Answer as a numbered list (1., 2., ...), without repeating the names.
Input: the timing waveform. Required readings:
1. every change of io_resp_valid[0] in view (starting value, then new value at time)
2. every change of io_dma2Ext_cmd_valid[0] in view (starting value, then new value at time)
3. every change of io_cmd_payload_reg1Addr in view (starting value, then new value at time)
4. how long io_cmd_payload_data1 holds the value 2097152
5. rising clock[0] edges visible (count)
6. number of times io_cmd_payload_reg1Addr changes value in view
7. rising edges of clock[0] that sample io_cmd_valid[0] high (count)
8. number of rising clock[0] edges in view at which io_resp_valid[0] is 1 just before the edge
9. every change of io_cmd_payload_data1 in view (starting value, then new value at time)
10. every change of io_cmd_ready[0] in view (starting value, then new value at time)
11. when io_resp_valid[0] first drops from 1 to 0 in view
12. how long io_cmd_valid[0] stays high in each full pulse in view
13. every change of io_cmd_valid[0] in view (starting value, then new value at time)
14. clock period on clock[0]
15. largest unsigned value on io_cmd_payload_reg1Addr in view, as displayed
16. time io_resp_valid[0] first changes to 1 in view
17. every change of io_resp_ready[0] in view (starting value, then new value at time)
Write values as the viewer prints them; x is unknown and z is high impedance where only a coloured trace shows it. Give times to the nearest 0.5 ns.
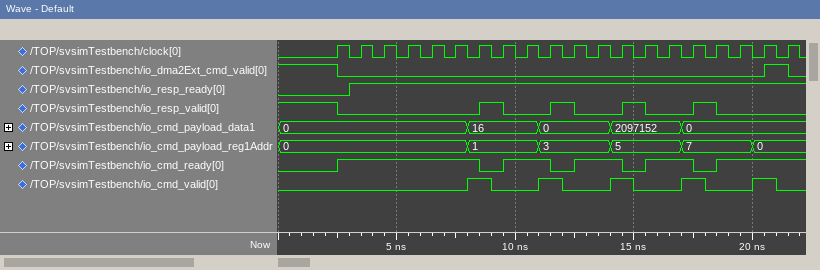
1. 1, 0 at 2.5 ns, 1 at 8.5 ns, 0 at 9.5 ns, 1 at 11.5 ns, 0 at 12.5 ns, 1 at 14.5 ns, 0 at 15.5 ns, 1 at 17.5 ns, 0 at 18.5 ns
2. 1, 0 at 2.5 ns, 1 at 20.5 ns, 0 at 21.5 ns
3. 0, 1 at 8 ns, 3 at 11 ns, 5 at 14 ns, 7 at 17 ns, 0 at 20 ns
4. 3 ns
5. 20
6. 5
7. 5
8. 5
9. 0, 16 at 8 ns, 0 at 11 ns, 2097152 at 14 ns, 0 at 17 ns
10. 0, 1 at 2.5 ns, 0 at 8.5 ns, 1 at 9.5 ns, 0 at 11.5 ns, 1 at 12.5 ns, 0 at 14.5 ns, 1 at 15.5 ns, 0 at 17.5 ns, 1 at 18.5 ns
11. 2.5 ns
12. 1 ns, 1 ns, 1 ns, 1 ns, 1 ns
13. 0, 1 at 8 ns, 0 at 9 ns, 1 at 11 ns, 0 at 12 ns, 1 at 14 ns, 0 at 15 ns, 1 at 17 ns, 0 at 18 ns, 1 at 20 ns, 0 at 21 ns
14. 1 ns
15. 7
16. 8.5 ns
17. 0, 1 at 3 ns
